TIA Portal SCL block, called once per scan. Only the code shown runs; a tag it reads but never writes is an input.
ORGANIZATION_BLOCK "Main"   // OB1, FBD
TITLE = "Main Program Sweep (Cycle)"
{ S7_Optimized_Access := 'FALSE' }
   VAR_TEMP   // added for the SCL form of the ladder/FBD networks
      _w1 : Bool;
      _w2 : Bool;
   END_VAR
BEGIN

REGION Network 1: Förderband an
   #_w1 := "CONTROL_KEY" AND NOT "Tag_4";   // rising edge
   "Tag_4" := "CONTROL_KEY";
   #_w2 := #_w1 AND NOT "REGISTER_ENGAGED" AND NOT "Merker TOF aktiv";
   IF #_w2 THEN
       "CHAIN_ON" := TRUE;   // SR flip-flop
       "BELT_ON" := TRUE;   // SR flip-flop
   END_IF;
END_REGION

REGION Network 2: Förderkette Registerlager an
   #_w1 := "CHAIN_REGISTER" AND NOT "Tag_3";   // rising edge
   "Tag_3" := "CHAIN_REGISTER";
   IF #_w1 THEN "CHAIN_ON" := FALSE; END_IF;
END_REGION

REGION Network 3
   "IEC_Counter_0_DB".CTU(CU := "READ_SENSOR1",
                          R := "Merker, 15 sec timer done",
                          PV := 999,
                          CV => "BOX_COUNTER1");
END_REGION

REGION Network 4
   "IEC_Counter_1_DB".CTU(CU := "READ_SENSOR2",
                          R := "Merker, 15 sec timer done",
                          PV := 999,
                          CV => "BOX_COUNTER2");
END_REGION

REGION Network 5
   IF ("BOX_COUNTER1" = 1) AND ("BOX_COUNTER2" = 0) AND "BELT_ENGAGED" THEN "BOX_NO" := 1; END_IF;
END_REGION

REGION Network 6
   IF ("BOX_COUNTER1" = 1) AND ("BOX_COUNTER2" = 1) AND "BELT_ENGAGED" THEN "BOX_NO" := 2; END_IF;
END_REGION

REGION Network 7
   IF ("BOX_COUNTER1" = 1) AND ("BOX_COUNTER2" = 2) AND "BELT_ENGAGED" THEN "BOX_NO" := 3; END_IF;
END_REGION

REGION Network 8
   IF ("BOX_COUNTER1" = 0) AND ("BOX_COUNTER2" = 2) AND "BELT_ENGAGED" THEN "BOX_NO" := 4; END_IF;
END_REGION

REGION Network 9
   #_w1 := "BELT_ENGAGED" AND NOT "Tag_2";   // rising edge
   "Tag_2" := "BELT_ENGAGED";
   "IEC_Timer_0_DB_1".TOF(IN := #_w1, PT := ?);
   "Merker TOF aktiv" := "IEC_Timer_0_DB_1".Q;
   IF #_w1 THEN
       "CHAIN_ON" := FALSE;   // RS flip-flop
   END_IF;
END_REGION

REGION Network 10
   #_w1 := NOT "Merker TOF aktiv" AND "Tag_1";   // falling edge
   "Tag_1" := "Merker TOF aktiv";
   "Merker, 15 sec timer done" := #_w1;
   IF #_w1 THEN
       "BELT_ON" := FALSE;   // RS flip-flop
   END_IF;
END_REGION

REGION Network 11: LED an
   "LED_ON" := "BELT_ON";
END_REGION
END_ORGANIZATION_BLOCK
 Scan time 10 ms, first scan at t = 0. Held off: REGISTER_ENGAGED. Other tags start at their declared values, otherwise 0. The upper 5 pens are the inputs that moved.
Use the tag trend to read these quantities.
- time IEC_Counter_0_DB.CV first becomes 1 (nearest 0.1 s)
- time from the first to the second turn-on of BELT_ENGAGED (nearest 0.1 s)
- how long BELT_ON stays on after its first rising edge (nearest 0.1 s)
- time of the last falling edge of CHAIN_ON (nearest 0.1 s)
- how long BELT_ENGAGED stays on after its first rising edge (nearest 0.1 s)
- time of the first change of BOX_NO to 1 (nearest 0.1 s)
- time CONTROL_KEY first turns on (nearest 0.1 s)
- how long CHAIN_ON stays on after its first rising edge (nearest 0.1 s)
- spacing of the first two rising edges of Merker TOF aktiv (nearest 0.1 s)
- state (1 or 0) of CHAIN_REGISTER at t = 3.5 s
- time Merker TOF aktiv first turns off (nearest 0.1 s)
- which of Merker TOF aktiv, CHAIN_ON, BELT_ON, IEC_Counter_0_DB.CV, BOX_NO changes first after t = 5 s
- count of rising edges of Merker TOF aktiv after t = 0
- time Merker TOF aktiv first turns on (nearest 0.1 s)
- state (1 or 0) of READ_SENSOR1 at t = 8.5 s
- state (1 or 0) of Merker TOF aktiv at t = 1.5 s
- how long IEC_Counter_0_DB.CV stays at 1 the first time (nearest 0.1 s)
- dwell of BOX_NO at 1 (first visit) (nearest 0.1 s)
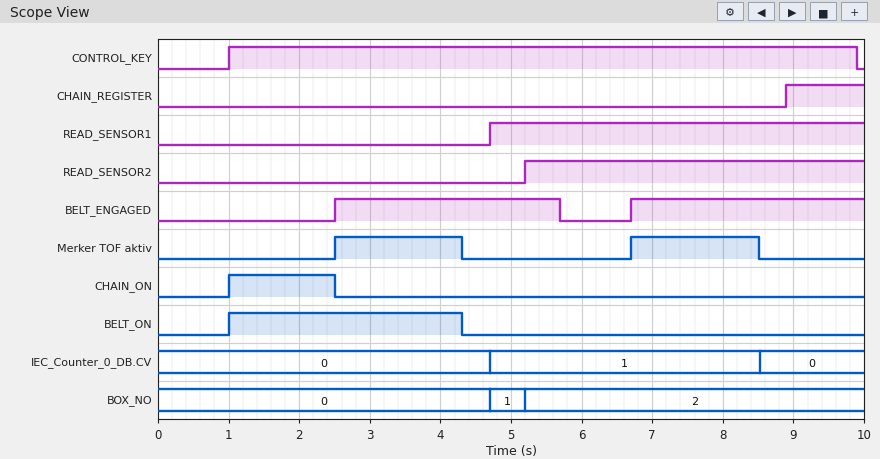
4.7 s
4.2 s
3.3 s
2.5 s
3.2 s
4.7 s
1.0 s
1.5 s
4.2 s
0
4.3 s
BOX_NO
2
2.5 s
1
0
3.8 s
0.5 s
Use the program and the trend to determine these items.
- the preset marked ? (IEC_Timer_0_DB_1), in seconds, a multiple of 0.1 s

1.8 s
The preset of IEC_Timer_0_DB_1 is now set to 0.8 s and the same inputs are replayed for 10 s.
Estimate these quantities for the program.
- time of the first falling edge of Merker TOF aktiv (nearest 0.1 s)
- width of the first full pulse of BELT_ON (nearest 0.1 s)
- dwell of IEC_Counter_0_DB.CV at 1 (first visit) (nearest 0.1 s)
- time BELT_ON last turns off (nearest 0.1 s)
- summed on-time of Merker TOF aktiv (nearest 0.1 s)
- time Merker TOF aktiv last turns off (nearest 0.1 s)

3.3 s
2.3 s
2.8 s
3.3 s
1.6 s
7.5 s
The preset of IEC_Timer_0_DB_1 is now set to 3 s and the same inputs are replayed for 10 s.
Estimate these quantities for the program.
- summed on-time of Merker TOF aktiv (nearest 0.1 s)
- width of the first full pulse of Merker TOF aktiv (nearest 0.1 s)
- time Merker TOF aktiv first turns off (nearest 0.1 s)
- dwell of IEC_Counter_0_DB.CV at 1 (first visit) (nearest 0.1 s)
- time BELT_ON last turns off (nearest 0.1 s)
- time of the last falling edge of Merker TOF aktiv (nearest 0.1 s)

6.0 s
3.0 s
5.5 s
0.8 s
5.5 s
9.7 s
